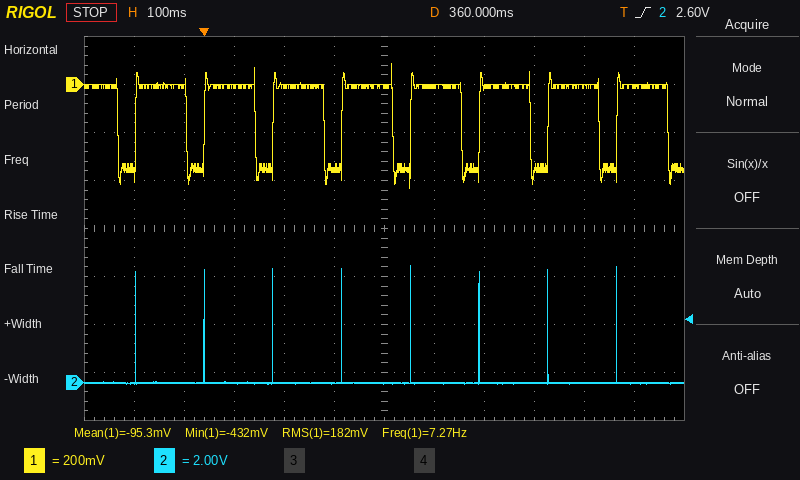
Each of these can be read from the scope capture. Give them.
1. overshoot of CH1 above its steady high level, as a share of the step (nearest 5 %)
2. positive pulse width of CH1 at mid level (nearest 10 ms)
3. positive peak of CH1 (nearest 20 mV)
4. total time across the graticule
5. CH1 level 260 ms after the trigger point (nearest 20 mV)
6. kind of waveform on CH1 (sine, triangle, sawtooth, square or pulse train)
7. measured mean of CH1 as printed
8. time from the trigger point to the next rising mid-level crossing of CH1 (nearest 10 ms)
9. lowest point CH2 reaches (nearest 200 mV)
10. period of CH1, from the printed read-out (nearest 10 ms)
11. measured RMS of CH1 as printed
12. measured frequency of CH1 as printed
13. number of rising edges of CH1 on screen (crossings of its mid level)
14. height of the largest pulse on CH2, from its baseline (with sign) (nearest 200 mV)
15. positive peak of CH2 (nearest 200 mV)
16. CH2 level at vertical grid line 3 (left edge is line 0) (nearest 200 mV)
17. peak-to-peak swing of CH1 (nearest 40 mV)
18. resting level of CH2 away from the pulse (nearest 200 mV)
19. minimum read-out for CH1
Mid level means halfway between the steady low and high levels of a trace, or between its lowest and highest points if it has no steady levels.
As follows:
30 %
100 ms
80 mV
1.2 s
-340 mV
pulse train
-95.3 mV
140 ms
0.0 V
140 ms
182 mV
7.27 Hz
8
+4.8 V
4.8 V
0.0 V
520 mV
0.0 V
-432 mV
